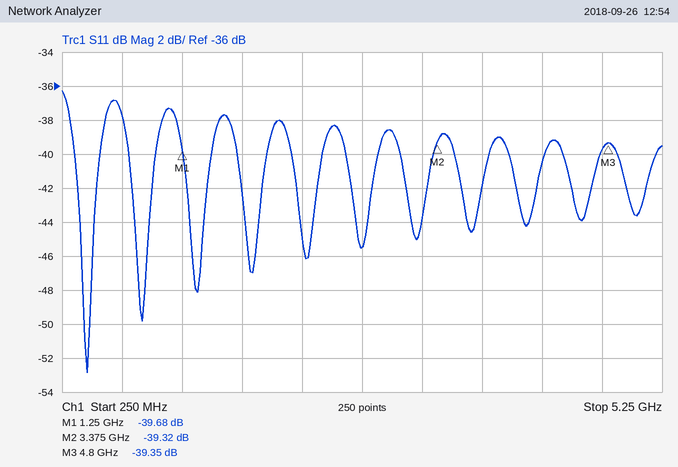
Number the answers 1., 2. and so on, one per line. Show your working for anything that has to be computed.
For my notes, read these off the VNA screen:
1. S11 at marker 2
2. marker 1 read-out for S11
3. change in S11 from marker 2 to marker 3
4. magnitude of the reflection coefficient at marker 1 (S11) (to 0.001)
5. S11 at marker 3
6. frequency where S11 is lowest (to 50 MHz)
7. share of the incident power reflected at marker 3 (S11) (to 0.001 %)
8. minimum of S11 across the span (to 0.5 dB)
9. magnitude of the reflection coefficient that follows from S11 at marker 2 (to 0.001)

1. -39.32 dB
2. -39.68 dB
3. -39.35 − (-39.32) = -0.03 dB
4. 10^(-39.68/20) ≈ 0.010
5. -39.35 dB
6. 450 MHz
7. 10^(-39.35/10) ≈ 0.012 %
8. -53.0 dB
9. 10^(-39.32/20) ≈ 0.011
